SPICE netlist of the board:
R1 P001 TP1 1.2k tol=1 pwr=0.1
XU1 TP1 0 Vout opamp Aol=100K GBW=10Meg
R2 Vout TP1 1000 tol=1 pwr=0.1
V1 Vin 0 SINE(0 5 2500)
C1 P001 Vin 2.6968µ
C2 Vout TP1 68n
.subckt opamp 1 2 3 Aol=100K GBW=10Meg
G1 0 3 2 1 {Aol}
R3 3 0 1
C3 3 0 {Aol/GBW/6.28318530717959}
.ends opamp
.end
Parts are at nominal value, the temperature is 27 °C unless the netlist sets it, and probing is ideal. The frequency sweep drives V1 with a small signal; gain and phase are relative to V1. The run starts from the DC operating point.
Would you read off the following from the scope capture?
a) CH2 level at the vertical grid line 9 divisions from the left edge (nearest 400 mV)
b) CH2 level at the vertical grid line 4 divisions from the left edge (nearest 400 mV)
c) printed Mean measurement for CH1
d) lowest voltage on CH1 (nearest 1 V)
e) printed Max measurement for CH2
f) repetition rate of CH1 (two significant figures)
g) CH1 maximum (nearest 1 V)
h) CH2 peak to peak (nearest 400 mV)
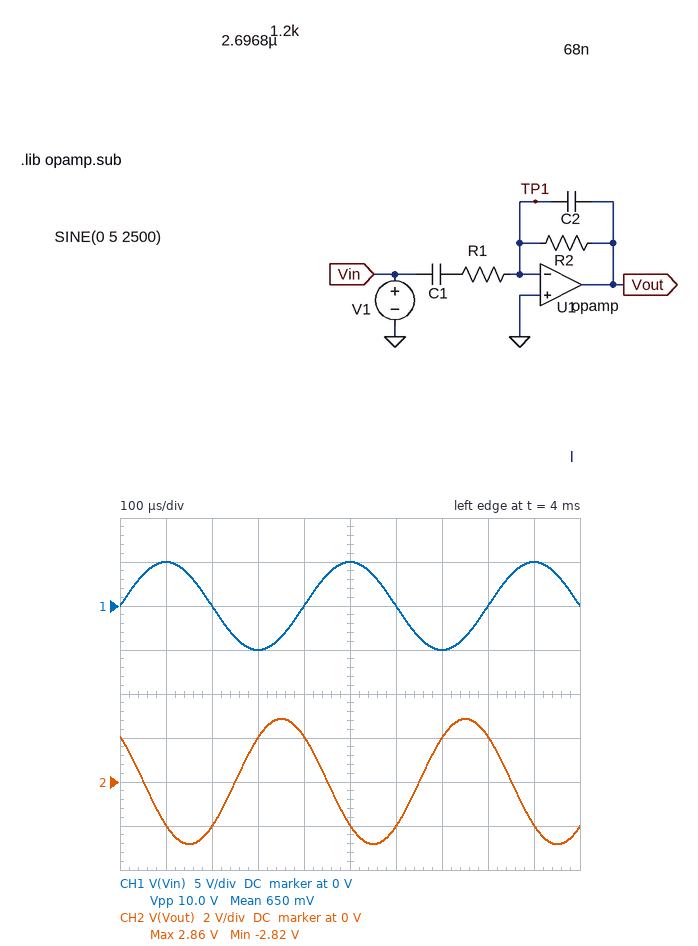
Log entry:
-2.0 V
2.0 V
650 mV
-5 V
2.86 V
2.5 kHz
5 V
5.6 V
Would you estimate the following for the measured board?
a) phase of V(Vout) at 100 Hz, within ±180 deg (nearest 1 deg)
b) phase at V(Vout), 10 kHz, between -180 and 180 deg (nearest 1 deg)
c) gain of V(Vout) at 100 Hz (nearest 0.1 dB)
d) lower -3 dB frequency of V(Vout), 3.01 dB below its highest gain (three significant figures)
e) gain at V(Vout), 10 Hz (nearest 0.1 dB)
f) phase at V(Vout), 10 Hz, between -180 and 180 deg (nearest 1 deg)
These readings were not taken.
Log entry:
-156 deg
103 deg
-2.5 dB
47.2 Hz
-15.6 dB
-102 deg
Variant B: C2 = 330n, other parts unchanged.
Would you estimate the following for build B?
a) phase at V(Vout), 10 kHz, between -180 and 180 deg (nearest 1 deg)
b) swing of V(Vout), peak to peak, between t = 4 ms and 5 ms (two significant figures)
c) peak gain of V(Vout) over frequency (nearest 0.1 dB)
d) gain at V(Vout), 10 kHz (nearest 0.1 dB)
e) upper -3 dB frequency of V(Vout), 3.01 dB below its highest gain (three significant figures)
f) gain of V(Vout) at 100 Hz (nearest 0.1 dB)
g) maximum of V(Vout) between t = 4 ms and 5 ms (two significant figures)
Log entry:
93 deg
1.6 V
-2.4 dB
-27.9 dB
573 Hz
-2.7 dB
810 mV
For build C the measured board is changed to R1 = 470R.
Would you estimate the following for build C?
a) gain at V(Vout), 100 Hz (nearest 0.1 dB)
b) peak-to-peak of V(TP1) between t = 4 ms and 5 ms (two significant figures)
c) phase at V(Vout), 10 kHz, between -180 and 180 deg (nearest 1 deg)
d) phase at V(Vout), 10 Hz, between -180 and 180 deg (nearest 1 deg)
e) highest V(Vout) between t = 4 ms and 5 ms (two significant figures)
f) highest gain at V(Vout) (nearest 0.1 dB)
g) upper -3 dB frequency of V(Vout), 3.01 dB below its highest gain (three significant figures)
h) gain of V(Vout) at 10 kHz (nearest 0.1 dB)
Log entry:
2.4 dB
3.6 mV
104 deg
-95 deg
7.3 V
6.1 dB
2.58 kHz
-6.3 dB
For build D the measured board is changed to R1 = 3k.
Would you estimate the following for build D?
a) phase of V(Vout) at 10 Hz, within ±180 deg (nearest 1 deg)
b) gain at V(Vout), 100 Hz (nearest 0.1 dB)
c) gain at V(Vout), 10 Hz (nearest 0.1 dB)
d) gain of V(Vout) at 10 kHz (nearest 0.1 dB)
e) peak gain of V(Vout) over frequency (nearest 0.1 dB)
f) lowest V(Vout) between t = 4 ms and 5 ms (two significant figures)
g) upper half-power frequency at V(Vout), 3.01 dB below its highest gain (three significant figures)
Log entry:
-117 deg
-9.7 dB
-16.4 dB
-22.4 dB
-9.6 dB
-1.1 V
2.38 kHz
